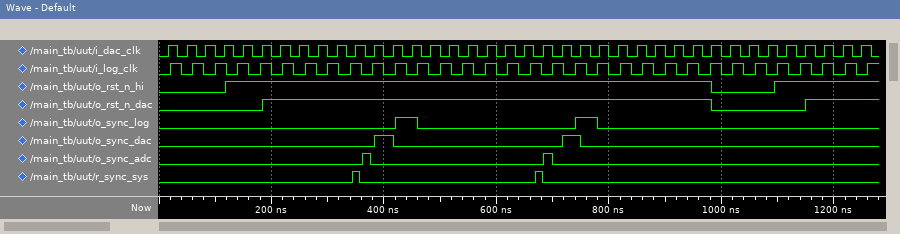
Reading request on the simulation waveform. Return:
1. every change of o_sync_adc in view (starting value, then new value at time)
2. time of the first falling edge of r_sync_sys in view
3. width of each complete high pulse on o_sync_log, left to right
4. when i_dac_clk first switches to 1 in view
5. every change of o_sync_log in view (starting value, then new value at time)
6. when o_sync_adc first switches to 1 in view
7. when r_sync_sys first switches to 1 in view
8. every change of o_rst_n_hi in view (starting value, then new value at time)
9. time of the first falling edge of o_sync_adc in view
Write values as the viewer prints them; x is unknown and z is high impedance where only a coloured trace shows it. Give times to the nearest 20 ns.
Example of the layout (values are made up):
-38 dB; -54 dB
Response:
0, 1 at 360 ns, 0 at 380 ns, 1 at 680 ns, 0 at 700 ns; 360 ns; 40 ns, 40 ns; 20 ns; 0, 1 at 420 ns, 0 at 460 ns, 1 at 740 ns, 0 at 780 ns; 360 ns; 340 ns; 0, 1 at 120 ns, 0 at 980 ns, 1 at 1100 ns; 380 ns
